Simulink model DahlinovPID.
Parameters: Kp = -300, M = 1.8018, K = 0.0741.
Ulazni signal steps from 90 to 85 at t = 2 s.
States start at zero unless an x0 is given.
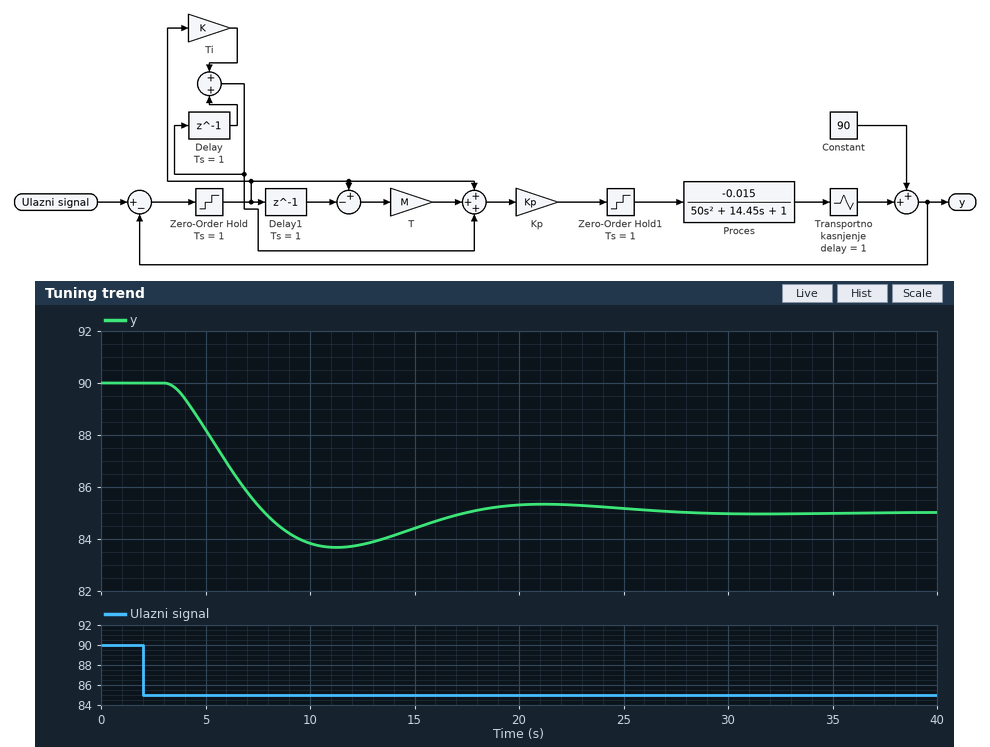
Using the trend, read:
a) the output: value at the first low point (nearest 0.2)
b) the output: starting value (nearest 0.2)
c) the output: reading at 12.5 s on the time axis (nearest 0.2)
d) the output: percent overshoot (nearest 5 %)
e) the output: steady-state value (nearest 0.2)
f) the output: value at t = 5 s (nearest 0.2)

83.6
90.0
83.8
25 %
85.0
88.2
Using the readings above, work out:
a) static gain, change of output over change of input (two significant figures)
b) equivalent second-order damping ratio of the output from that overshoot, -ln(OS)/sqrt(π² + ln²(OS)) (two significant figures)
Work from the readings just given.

1.0
0.40
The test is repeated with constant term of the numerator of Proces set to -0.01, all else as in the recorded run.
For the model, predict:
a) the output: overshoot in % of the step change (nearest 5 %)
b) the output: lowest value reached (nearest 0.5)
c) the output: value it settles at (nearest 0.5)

15 %
84.5
85.0
